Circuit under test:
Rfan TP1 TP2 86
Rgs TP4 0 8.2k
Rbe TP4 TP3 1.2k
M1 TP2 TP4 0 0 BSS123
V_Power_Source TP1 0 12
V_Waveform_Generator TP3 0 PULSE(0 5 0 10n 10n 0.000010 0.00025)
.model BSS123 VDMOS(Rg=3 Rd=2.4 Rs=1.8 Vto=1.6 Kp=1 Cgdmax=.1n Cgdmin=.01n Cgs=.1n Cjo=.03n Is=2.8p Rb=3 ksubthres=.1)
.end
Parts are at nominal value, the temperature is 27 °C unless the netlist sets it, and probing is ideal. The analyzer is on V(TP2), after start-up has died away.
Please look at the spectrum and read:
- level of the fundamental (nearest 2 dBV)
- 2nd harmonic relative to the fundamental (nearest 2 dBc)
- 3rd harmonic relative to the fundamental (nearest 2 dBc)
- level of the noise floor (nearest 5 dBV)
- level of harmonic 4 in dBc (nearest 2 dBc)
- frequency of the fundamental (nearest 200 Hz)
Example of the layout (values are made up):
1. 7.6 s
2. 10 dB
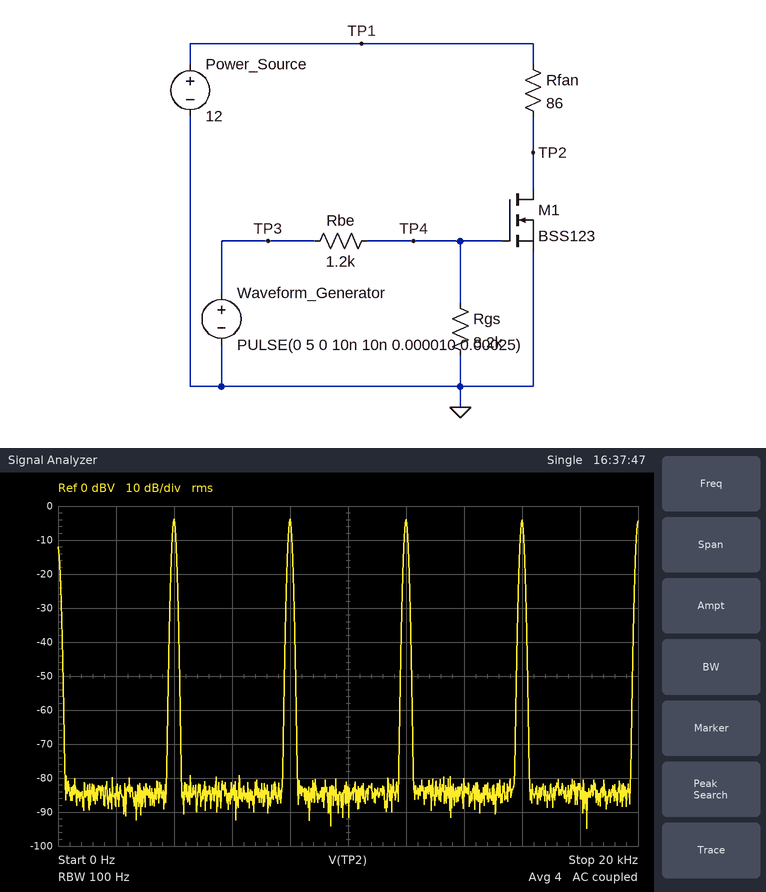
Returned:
1. -4 dBV
2. 0 dBc
3. 0 dBc
4. -85 dBV
5. 0 dBc
6. 4.0 kHz
